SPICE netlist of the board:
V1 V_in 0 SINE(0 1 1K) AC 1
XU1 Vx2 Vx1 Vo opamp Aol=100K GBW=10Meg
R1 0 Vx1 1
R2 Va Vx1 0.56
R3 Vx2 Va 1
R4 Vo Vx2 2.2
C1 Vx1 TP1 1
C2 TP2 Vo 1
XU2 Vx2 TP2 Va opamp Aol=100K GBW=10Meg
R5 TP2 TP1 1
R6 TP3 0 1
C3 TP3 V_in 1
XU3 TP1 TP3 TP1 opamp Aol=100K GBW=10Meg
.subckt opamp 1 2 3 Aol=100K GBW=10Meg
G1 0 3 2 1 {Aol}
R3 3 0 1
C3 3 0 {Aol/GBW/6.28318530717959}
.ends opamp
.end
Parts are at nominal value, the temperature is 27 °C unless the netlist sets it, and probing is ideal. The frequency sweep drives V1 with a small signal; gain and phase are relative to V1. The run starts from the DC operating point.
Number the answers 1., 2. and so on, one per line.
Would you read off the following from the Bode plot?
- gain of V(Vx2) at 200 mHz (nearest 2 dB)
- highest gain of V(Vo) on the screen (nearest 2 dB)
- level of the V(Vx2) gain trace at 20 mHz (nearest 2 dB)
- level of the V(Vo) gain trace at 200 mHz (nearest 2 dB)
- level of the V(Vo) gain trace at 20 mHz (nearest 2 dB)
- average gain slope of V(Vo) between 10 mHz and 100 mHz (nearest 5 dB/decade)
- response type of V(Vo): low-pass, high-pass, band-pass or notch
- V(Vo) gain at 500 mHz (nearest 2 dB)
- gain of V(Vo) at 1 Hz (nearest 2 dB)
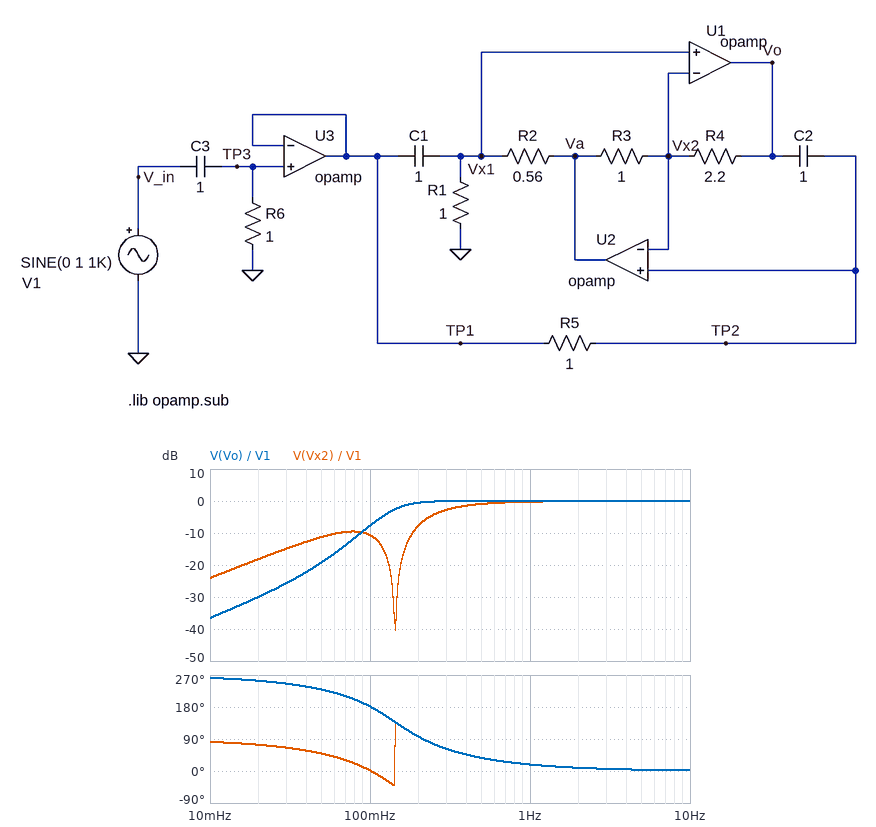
1. -8 dB
2. 0 dB
3. -18 dB
4. 0 dB
5. -30 dB
6. 30 dB/decade
7. high-pass
8. 0 dB
9. 0 dB
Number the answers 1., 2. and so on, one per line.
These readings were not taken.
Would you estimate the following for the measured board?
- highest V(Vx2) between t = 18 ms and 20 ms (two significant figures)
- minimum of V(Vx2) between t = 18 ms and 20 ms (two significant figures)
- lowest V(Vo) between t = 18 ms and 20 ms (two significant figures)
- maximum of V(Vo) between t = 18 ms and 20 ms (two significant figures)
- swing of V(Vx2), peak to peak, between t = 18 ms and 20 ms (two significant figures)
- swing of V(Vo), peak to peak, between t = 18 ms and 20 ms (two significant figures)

1. 1.0 V
2. -1.0 V
3. -1.0 V
4. 1.0 V
5. 2.0 V
6. 2.0 V
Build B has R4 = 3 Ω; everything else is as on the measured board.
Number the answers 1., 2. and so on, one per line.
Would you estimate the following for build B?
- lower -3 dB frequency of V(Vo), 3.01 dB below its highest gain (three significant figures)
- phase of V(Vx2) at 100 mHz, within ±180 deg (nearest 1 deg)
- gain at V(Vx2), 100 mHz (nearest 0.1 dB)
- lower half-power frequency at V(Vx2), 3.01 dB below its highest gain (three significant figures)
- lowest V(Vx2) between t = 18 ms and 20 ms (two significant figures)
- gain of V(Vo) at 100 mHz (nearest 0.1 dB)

1. 109 mHz
2. -14 deg
3. -15.8 dB
4. 278 mHz
5. -1.0 V
6. -3.8 dB
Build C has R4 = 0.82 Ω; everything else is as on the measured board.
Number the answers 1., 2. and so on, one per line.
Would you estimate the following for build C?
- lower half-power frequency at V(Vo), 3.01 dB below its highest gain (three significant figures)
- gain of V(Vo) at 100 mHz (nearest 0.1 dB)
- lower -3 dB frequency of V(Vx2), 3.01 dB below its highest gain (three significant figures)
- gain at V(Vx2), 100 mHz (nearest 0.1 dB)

1. 254 mHz
2. -13.1 dB
3. 352 mHz
4. -6.0 dB
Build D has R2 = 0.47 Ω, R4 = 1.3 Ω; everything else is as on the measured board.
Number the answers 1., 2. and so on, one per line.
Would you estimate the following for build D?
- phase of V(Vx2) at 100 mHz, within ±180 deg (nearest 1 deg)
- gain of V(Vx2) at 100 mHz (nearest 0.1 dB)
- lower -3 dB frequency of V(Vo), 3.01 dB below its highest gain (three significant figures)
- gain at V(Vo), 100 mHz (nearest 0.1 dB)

1. 31 deg
2. -6.5 dB
3. 216 mHz
4. -20.7 dB
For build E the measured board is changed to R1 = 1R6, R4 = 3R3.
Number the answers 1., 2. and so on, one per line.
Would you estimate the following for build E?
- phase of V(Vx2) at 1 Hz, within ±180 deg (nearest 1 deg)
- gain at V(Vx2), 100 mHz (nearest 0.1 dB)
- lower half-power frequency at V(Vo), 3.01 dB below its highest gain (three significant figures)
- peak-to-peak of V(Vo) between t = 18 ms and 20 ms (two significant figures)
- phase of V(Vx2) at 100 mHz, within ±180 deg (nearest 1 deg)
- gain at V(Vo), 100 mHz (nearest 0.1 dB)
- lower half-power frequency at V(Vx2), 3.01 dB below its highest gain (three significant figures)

1. 15 deg
2. -14.6 dB
3. 108 mHz
4. 2.0 V
5. -12 deg
6. -4.3 dB
7. 229 mHz
